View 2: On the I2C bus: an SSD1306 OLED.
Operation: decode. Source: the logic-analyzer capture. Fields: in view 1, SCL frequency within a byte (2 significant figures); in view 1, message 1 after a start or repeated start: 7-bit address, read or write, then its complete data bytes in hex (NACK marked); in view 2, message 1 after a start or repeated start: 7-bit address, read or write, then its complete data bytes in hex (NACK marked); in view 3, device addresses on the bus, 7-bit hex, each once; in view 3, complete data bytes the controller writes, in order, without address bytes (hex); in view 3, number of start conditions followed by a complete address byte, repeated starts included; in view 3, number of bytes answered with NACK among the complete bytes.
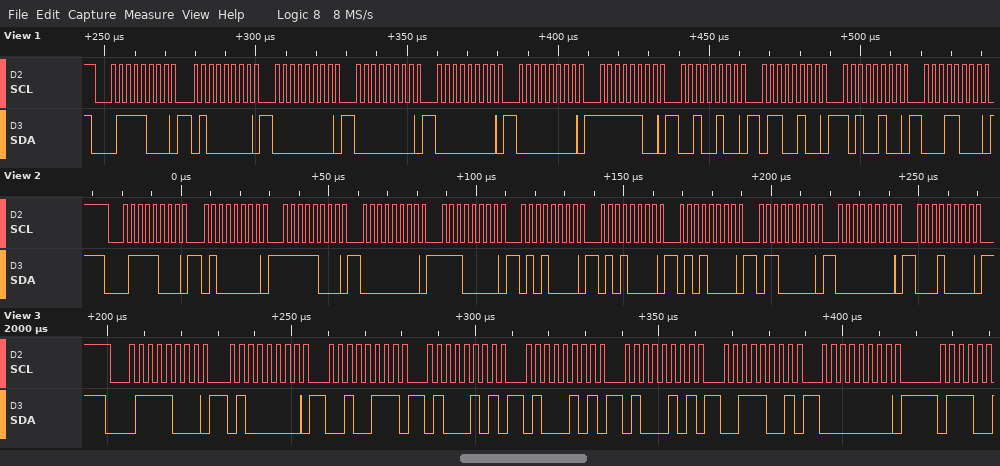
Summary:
400 kHz
0x3C write: 40 00 00 00 00 FC 24 64 A4 18
0x3C write: 40 F8 00 E0 50 50 50 60 00 10
0x3C
40 27 45 45 45 39 00
1
0
